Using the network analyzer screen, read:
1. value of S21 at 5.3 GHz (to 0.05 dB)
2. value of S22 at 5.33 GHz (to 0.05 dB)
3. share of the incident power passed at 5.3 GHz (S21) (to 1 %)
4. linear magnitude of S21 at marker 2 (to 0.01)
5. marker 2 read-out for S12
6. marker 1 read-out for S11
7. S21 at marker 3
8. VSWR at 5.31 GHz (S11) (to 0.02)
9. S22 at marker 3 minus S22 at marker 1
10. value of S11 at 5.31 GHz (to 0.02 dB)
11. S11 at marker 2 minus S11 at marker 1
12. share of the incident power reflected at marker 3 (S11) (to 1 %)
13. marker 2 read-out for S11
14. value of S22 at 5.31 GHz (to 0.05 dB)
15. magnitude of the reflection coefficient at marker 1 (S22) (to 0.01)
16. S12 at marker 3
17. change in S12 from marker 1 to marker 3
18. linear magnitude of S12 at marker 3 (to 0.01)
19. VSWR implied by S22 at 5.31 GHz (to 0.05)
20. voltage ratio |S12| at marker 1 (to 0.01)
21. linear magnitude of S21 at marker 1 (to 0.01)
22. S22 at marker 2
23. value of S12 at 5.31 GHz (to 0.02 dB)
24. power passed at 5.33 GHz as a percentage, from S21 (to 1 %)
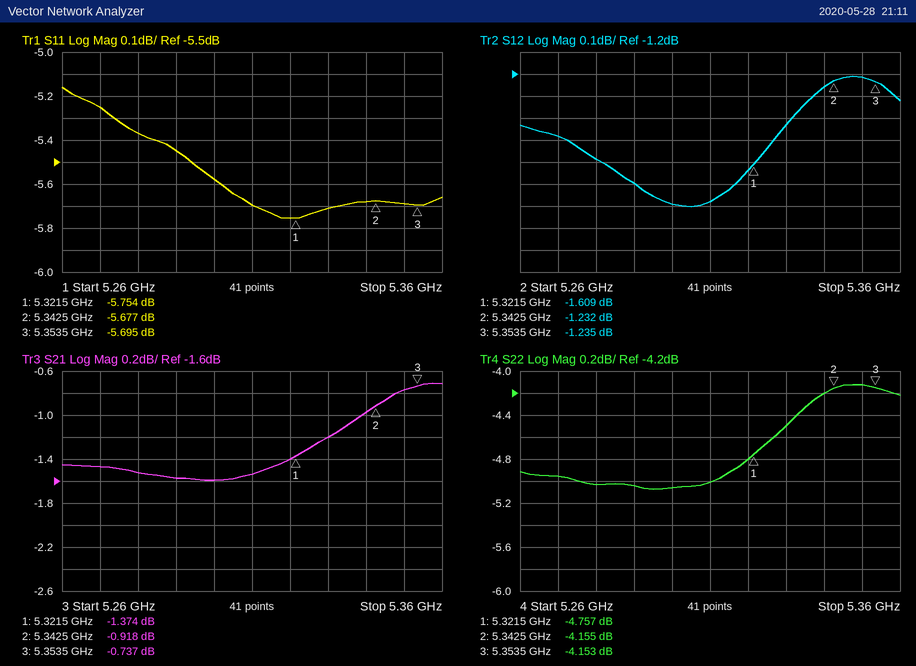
-1.60 dB
-4.50 dB
69 %
0.90
-1.232 dB
-5.754 dB
-0.737 dB
3.16
0.604 dB
-5.70 dB
0.077 dB
27 %
-5.677 dB
-5.00 dB
0.58
-1.235 dB
0.374 dB
0.87
3.55
0.83
0.85
-4.155 dB
-1.78 dB
76 %
